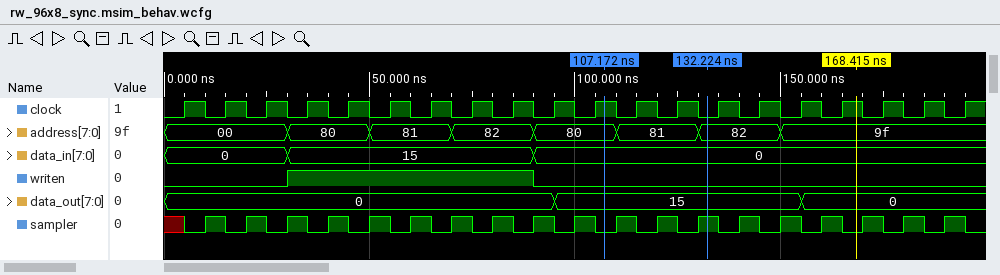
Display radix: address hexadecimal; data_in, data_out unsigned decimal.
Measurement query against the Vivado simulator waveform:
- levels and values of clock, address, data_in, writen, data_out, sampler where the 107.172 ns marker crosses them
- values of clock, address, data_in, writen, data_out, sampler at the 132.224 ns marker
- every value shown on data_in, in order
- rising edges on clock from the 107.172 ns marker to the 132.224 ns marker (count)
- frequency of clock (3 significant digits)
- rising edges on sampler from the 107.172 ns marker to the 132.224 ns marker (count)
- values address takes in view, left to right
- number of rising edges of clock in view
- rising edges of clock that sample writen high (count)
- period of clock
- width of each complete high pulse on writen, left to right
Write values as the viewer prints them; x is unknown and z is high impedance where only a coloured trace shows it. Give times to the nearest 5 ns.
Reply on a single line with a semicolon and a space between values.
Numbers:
clock=1, address=80, data_in=0, writen=0, data_out=15, sampler=0; clock=0, address=82, data_in=0, writen=0, data_out=15, sampler=1; 0, 15, 0; 2; 100 MHz; 3; 00, 80, 81, 82, 80, 81, 82, 9f; 20; 6; 10 ns; 60 ns
